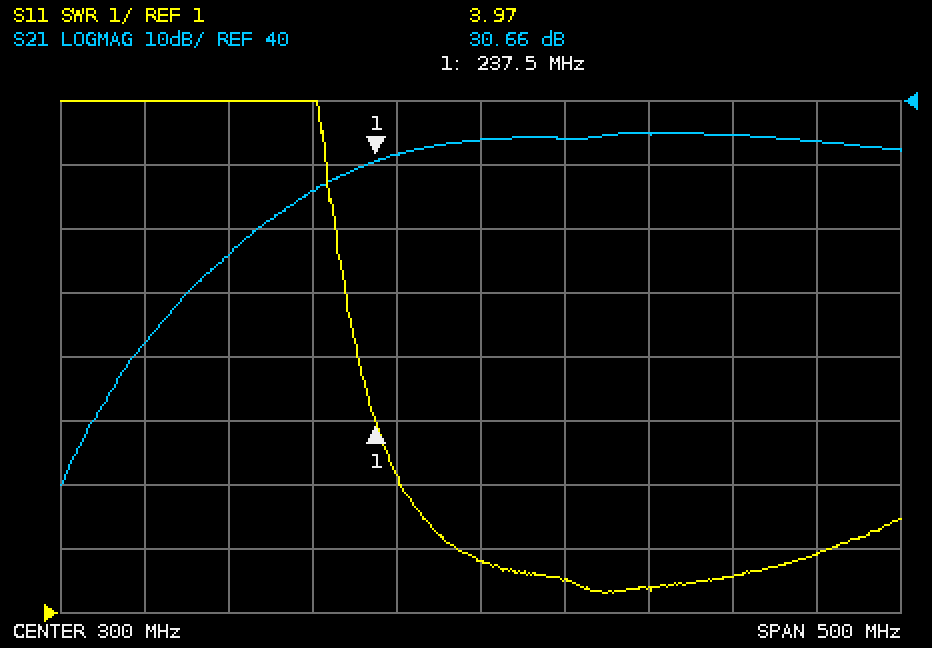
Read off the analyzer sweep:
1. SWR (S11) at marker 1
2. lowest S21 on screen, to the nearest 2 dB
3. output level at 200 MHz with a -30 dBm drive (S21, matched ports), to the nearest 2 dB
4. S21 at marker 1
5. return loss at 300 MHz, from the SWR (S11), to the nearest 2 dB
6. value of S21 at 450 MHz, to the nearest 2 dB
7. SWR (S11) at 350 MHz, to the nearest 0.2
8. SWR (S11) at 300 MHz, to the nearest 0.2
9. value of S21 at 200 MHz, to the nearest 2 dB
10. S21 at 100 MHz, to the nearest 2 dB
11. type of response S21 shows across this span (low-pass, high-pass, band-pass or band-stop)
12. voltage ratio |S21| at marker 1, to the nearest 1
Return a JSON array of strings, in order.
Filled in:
["3.97", "-20 dB", "-4 dBm", "30.66 dB", "10 dB", "34 dB", "1.6", "1.8", "26 dB", "2 dB", "high-pass", "34"]
